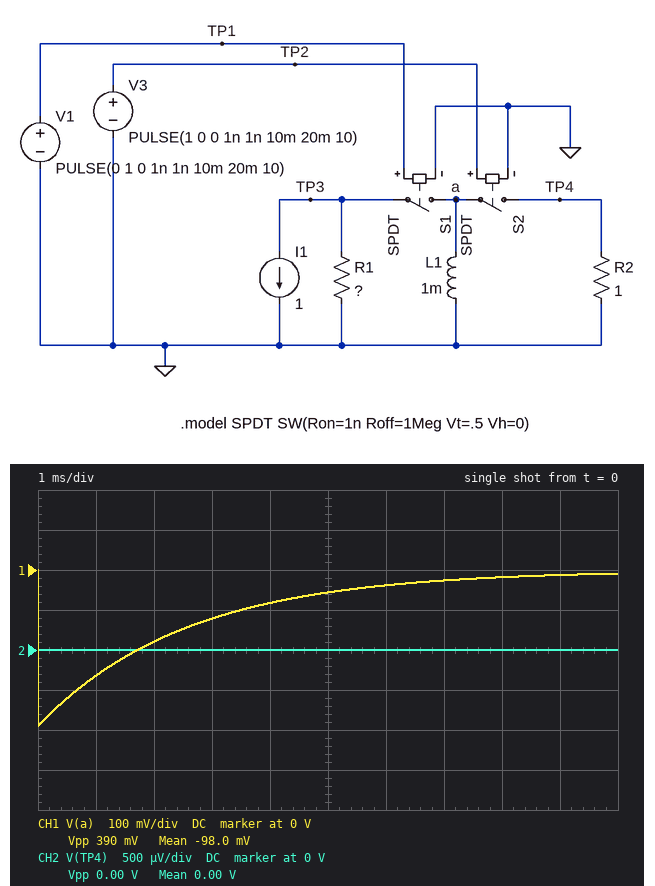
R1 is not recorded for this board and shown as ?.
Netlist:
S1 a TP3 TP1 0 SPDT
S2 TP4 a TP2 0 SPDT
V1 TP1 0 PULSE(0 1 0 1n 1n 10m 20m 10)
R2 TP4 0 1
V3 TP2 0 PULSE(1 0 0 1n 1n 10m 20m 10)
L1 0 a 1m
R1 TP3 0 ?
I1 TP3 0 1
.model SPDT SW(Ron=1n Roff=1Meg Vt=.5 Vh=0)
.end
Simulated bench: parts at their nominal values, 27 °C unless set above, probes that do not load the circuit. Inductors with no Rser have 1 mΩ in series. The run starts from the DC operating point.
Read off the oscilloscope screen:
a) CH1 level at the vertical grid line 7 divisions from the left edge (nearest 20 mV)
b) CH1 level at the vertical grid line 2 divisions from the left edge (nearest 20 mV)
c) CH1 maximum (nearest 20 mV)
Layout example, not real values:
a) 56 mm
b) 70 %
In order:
a) -20 mV
b) -180 mV
c) 0 V
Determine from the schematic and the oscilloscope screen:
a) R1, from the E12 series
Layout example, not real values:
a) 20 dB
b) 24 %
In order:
a) 0.39 Ω
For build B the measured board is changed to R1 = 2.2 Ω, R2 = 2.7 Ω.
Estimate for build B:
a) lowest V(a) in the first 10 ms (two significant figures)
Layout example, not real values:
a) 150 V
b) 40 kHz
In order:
a) -2.2 V
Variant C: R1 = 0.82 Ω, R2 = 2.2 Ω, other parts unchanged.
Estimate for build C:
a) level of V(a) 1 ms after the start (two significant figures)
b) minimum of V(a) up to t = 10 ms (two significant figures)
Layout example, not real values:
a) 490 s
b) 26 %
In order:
a) -360 mV
b) -820 mV
